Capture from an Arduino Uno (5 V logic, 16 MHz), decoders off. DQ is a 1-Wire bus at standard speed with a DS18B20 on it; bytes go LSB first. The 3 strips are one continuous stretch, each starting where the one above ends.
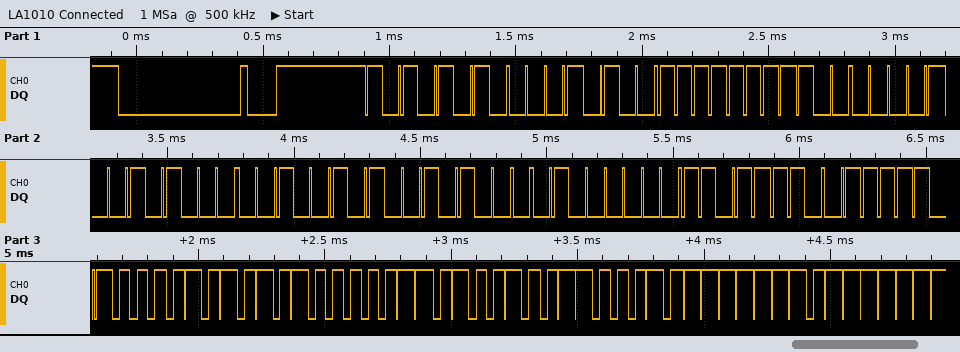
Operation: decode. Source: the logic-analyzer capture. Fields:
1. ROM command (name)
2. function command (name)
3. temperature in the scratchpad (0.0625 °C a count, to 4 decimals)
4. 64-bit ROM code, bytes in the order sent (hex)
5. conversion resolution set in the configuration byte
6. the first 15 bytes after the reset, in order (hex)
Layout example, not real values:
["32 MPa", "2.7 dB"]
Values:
["Match ROM", "Read Scratchpad", "85.0000 °C", "28 FF 81 14 A4 14 02 7B", "12 bits", "55 28 FF 81 14 A4 14 02 7B BE 50 05 4B 46 7F"]
